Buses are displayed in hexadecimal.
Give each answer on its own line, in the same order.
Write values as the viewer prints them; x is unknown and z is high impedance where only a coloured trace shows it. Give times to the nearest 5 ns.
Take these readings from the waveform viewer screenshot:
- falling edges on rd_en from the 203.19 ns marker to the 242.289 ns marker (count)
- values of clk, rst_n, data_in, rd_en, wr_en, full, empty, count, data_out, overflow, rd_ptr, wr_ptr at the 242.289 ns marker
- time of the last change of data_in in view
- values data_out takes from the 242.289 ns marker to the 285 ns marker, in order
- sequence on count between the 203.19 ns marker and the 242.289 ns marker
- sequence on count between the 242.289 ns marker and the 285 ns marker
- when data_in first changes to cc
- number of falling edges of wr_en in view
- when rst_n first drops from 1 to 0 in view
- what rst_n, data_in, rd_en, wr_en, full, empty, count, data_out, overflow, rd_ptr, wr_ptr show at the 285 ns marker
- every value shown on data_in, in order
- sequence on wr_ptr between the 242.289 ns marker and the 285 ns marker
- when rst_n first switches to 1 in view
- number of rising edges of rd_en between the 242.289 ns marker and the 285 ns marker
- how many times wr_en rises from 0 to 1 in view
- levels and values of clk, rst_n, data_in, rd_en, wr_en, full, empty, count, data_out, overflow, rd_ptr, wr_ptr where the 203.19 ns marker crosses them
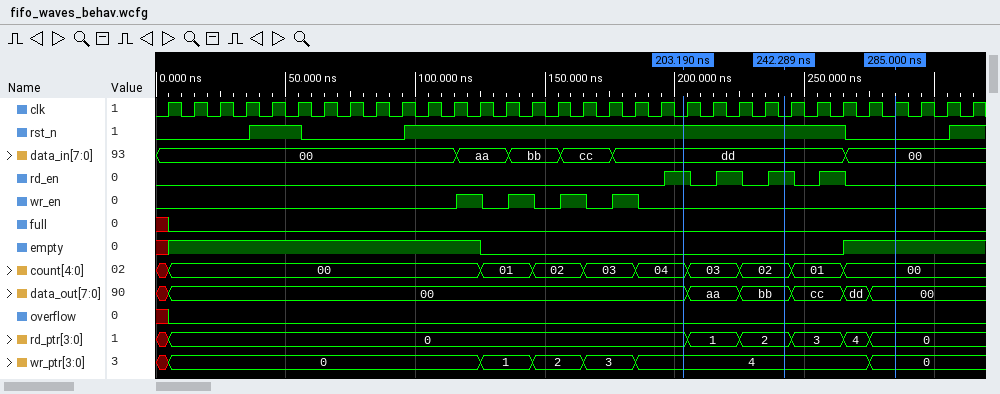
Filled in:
2
clk=0, rst_n=1, data_in=dd, rd_en=1, wr_en=0, full=0, empty=0, count=02, data_out=bb, overflow=0, rd_ptr=2, wr_ptr=4
265 ns
bb, cc, dd, 00
04, 03, 02
02, 01, 00
155 ns
4
55 ns
rst_n=0, data_in=00, rd_en=0, wr_en=0, full=0, empty=1, count=00, data_out=00, overflow=0, rd_ptr=0, wr_ptr=0
00, aa, bb, cc, dd, 00
4, 0
35 ns
1
4
clk=0, rst_n=1, data_in=dd, rd_en=1, wr_en=0, full=0, empty=0, count=04, data_out=00, overflow=0, rd_ptr=0, wr_ptr=4
